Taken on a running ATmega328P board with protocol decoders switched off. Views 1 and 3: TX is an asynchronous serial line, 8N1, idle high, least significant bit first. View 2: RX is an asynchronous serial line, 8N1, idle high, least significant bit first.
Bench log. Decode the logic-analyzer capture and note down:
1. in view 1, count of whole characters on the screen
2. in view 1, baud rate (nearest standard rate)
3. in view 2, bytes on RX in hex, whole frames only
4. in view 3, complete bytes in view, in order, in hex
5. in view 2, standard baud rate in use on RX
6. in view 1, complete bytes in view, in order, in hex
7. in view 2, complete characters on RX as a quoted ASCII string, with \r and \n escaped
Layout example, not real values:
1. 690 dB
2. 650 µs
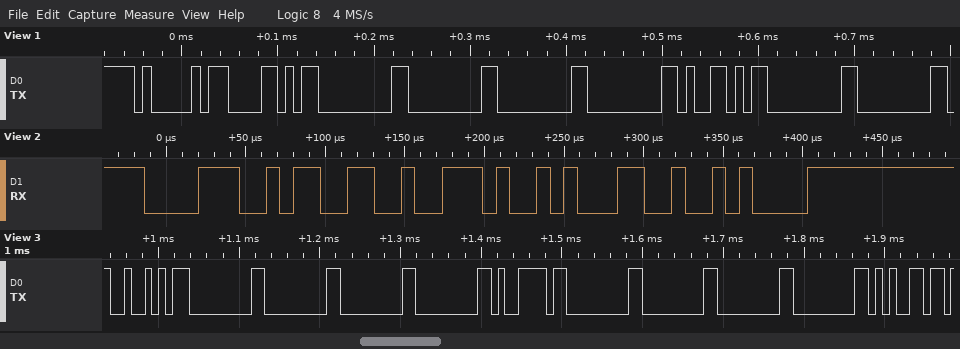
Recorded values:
1. 9
2. 115200 baud
3. 38 33 2E 31 0A
4. 0x52 0x00 0x00 0x00 0x00 0x79 0x00 0x00 0x00 0x00 0x65
5. 115200 baud
6. 41 58 00 00 00 00 59 00 00
7. "83.1\n"
